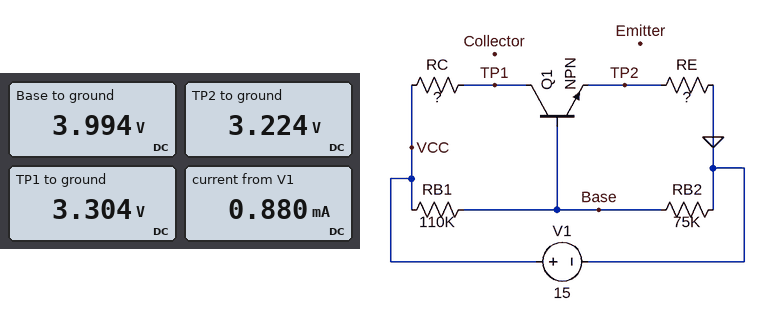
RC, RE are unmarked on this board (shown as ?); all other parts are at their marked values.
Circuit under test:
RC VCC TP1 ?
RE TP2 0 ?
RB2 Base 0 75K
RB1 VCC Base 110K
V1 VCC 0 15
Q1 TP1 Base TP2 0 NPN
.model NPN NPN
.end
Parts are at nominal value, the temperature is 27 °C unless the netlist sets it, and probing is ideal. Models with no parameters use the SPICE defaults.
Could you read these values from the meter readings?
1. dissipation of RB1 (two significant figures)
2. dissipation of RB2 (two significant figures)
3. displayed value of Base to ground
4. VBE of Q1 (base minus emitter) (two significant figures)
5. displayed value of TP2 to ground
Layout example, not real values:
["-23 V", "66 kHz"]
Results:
["1.1 mW", "210 µW", "3.994 V", "770 mV", "3.224 V"]
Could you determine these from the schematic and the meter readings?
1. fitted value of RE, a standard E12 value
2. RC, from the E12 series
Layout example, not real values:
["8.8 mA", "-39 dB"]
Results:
["3.9 kΩ", "15 kΩ"]
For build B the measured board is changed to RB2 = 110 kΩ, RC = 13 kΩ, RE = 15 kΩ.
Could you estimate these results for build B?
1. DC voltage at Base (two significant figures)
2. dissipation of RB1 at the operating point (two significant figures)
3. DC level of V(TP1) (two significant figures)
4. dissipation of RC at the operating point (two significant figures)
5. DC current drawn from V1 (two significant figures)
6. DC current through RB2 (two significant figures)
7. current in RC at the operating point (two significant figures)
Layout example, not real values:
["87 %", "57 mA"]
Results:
["7.3 V", "540 µW", "9.4 V", "2.4 mW", "500 µA", "66 µA", "430 µA"]
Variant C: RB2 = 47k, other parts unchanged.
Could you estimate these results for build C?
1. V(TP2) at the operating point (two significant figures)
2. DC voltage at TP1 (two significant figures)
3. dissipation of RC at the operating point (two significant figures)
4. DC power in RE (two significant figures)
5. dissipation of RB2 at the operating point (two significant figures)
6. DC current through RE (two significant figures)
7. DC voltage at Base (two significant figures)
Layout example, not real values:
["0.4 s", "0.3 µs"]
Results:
["3.1 V", "3.2 V", "9.2 mW", "2.5 mW", "320 µW", "800 µA", "3.9 V"]
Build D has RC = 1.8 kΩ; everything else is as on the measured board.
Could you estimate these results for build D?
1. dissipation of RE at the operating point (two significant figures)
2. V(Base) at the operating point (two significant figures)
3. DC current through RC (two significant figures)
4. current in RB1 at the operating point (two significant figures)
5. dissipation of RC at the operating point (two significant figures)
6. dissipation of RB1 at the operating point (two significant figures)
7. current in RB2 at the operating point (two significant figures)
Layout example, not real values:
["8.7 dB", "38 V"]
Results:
["5.8 mW", "5.5 V", "1.2 mA", "86 µA", "2.6 mW", "810 µW", "74 µA"]
